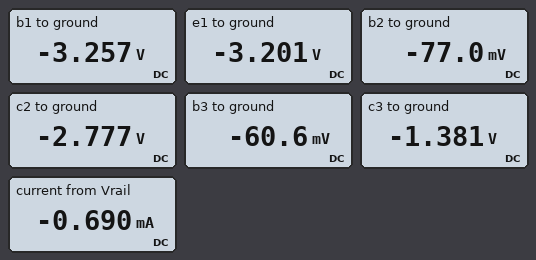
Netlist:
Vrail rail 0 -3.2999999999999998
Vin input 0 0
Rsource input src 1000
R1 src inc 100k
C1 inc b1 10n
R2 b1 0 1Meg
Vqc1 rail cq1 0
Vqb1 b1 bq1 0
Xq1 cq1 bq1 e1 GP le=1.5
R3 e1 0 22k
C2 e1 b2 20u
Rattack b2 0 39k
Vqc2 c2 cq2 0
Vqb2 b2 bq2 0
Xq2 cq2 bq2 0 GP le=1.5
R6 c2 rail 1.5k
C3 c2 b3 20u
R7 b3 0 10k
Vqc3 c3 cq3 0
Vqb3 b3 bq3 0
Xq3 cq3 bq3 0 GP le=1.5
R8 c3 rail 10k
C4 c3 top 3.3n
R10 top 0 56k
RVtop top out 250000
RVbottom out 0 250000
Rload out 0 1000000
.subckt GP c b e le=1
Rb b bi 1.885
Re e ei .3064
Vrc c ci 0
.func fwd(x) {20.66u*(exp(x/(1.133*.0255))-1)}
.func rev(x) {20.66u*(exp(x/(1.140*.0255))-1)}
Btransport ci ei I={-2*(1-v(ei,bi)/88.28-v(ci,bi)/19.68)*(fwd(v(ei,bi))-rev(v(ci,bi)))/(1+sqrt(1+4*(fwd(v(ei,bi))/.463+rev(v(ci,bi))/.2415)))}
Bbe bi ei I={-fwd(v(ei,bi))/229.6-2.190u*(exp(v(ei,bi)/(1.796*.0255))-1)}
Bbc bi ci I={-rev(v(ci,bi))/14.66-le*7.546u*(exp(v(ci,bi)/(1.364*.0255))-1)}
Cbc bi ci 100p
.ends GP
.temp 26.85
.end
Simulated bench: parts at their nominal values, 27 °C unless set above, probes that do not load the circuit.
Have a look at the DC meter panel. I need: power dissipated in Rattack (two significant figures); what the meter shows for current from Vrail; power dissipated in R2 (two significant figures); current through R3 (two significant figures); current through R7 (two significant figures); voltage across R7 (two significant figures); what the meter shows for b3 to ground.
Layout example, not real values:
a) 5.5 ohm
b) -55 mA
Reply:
a) 150 nW
b) -0.690 mA
c) 11 µW
d) 150 µA
e) 6.1 µA
f) 61 mV
g) -60.6 mV
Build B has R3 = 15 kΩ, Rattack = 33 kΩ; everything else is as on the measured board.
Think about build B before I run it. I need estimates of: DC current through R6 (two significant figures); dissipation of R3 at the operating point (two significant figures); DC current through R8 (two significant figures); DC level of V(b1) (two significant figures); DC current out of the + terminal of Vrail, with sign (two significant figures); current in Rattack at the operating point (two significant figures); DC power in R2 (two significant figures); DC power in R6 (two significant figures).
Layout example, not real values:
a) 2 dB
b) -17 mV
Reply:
a) 340 µA
b) 670 µW
c) 190 µA
d) -3.2 V
e) -740 µA
f) 2.3 µA
g) 10 µW
h) 170 µW
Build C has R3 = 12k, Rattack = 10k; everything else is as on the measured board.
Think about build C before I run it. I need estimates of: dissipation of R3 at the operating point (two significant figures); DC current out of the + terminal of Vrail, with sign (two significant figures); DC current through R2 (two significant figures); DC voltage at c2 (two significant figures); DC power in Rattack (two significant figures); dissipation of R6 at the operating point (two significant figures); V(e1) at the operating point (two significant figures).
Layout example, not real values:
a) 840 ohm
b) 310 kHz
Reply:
a) 800 µW
b) -660 µA
c) 3.2 µA
d) -3.0 V
e) 370 nW
f) 63 µW
g) -3.1 V
